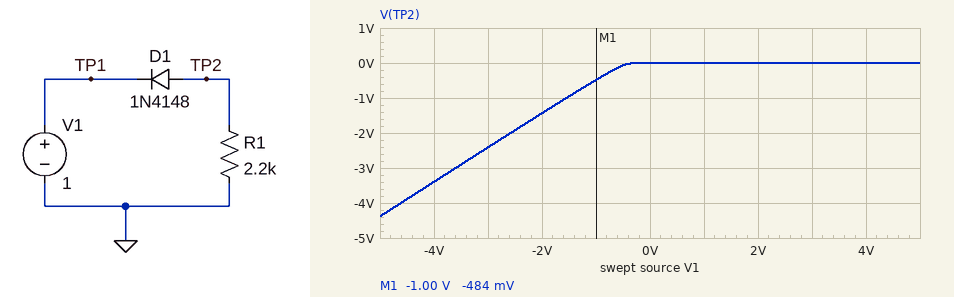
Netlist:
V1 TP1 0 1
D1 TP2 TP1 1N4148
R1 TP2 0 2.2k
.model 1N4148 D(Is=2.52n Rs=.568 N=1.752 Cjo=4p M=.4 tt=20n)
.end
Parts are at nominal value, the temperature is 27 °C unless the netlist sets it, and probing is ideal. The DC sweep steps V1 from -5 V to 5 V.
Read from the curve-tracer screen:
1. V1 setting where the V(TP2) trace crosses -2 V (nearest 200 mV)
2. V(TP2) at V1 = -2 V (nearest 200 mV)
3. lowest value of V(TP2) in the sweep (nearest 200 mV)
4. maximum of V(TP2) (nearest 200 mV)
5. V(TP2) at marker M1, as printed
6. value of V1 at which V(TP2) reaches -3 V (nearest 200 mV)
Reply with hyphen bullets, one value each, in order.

- -2.6 V
- -1.4 V
- -4.4 V
- 0 V
- -484 mV
- -3.6 V
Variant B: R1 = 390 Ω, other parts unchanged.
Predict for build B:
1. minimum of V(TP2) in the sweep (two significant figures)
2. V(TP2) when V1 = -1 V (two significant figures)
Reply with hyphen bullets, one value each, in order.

- -4.3 V
- -410 mV
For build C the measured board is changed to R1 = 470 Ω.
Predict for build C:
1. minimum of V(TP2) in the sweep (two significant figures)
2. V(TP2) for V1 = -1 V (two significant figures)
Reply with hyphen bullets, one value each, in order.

- -4.3 V
- -420 mV
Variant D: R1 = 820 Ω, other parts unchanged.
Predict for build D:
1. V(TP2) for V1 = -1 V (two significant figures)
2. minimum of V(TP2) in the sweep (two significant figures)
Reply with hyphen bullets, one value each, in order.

- -440 mV
- -4.3 V
